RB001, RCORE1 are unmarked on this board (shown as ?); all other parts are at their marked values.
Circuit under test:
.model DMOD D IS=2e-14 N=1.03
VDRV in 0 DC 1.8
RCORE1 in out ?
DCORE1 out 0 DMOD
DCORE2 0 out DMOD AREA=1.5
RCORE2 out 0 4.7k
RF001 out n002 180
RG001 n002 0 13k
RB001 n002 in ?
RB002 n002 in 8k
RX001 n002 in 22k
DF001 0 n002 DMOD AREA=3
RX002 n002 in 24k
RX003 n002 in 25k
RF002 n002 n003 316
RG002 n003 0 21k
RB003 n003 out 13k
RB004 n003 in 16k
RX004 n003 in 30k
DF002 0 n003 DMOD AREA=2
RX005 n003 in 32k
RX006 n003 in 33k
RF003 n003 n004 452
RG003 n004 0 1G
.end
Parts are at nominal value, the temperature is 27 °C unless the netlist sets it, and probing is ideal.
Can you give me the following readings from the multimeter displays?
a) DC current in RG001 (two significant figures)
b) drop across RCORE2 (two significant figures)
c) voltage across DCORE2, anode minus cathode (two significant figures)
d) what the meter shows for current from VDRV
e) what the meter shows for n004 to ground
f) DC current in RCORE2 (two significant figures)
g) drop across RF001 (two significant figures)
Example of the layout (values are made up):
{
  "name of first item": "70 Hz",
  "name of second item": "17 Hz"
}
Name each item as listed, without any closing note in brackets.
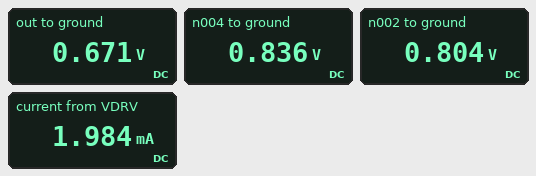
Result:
{
  "DC current in RG001": "62 µA",
  "drop across RCORE2": "670 mV",
  "voltage across DCORE2, anode minus cathode": "-670 mV",
  "what the meter shows for current from VDRV": "1.984 mA",
  "what the meter shows for n004 to ground": "0.836 V",
  "DC current in RCORE2": "140 µA",
  "drop across RF001": "130 mV"
}
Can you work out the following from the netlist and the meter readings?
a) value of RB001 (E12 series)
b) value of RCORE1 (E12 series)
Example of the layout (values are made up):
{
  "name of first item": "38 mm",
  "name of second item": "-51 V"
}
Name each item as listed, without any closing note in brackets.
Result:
{
  "value of RB001": "2.2 kΩ",
  "value of RCORE1": "1 kΩ"
}
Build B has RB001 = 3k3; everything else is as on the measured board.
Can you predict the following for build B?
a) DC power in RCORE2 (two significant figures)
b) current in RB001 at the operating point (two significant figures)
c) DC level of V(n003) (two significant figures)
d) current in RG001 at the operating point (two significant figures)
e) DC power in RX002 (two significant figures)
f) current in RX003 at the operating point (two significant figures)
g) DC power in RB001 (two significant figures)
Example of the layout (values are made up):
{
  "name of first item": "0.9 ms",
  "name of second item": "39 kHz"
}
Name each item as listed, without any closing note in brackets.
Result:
{
  "DC power in RCORE2": "95 µW",
  "current in RB001 at the operating point": "310 µA",
  "DC level of V(n003)": "810 mV",
  "current in RG001 at the operating point": "60 µA",
  "DC power in RX002": "43 µW",
  "current in RX003 at the operating point": "41 µA",
  "DC power in RB001": "320 µW"
}
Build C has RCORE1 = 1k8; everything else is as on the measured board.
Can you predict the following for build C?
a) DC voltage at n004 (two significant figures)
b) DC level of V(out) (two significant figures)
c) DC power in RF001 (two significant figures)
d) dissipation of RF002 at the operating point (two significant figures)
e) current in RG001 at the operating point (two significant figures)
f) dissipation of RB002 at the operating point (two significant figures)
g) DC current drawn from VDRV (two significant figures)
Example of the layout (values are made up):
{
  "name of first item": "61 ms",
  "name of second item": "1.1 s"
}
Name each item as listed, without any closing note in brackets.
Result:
{
  "DC voltage at n004": "830 mV",
  "DC level of V(out)": "660 mV",
  "DC power in RF001": "100 µW",
  "dissipation of RF002 at the operating point": "3.2 µW",
  "current in RG001 at the operating point": "61 µA",
  "dissipation of RB002 at the operating point": "130 µW",
  "DC current drawn from VDRV": "1.5 mA"
}
